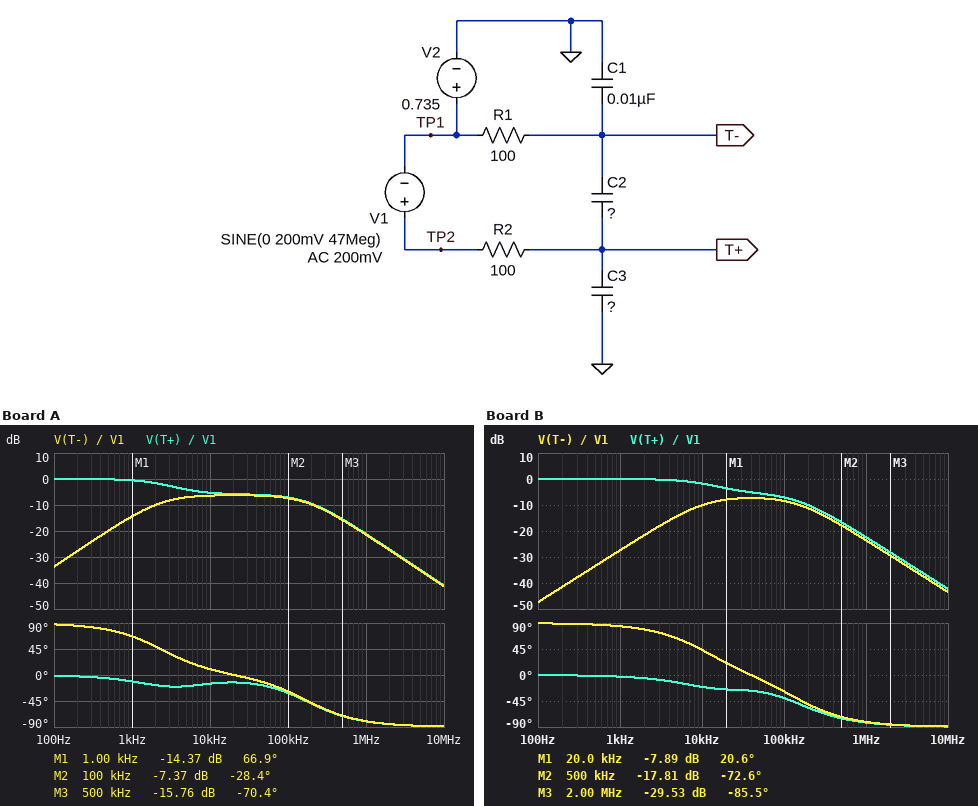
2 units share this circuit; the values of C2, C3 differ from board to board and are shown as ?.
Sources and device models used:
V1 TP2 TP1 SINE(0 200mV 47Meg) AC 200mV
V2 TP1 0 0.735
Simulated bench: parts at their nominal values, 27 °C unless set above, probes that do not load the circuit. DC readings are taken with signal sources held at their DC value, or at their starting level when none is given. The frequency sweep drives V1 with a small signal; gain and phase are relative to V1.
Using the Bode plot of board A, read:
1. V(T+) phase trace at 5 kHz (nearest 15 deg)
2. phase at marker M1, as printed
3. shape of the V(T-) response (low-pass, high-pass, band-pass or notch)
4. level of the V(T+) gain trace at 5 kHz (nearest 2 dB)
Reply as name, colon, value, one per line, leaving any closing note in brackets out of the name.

V(T+) phase trace at 5 kHz: -15 deg
phase at marker M1, as printed: 66.9 deg
shape of the V(T-) response: band-pass
level of the V(T+) gain trace at 5 kHz: -4 dB
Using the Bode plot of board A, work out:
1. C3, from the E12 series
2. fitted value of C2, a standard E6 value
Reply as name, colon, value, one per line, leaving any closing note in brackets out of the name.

C3, from the E12 series: 8.2 nF
fitted value of C2, a standard E6 value: 330 nF
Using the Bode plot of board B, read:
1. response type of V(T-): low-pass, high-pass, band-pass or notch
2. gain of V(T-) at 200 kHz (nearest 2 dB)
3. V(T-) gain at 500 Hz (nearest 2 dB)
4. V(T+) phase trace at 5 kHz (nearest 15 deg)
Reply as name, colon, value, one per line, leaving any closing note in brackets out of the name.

response type of V(T-): low-pass, high-pass, band-pass or notch: band-pass
gain of V(T-) at 200 kHz: -12 dB
V(T-) gain at 500 Hz: -34 dB
V(T+) phase trace at 5 kHz: -15 deg
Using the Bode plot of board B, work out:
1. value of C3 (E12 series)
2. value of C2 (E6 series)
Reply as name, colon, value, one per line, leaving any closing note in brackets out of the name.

value of C3: 12 nF
value of C2: 68 nF
